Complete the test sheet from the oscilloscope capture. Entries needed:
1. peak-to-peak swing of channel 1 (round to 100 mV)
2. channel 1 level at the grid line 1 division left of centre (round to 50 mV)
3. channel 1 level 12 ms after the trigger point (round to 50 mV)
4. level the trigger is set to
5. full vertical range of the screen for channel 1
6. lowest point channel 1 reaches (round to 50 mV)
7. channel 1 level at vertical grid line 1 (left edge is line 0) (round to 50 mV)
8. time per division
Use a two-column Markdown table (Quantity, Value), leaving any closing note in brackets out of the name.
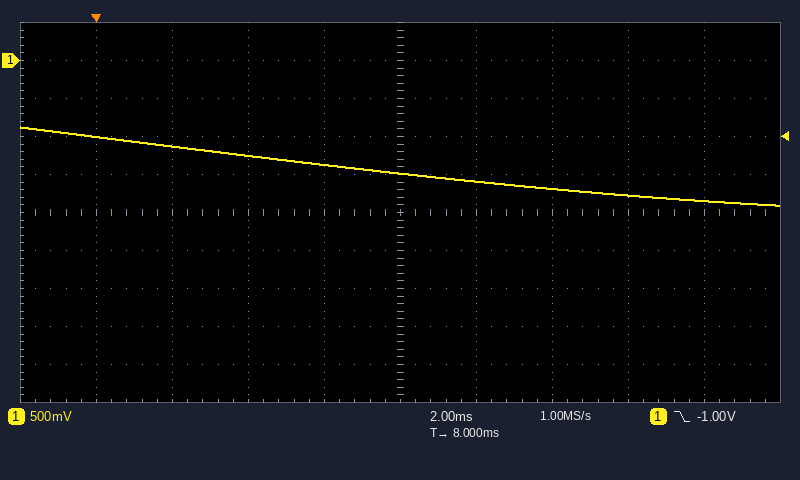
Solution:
| Quantity | Value |
|---|---|
| peak-to-peak swing of channel 1 | 1.00 V |
| channel 1 level at the grid line 1 division left of centre | -1.35 V |
| channel 1 level 12 ms after the trigger point | -1.70 V |
| level the trigger is set to | -1.00 V |
| full vertical range of the screen for channel 1 | 5 V |
| lowest point channel 1 reaches | -1.90 V |
| channel 1 level at vertical grid line 1 (left edge is line 0) | -1.00 V |
| time per division | 2 ms |
